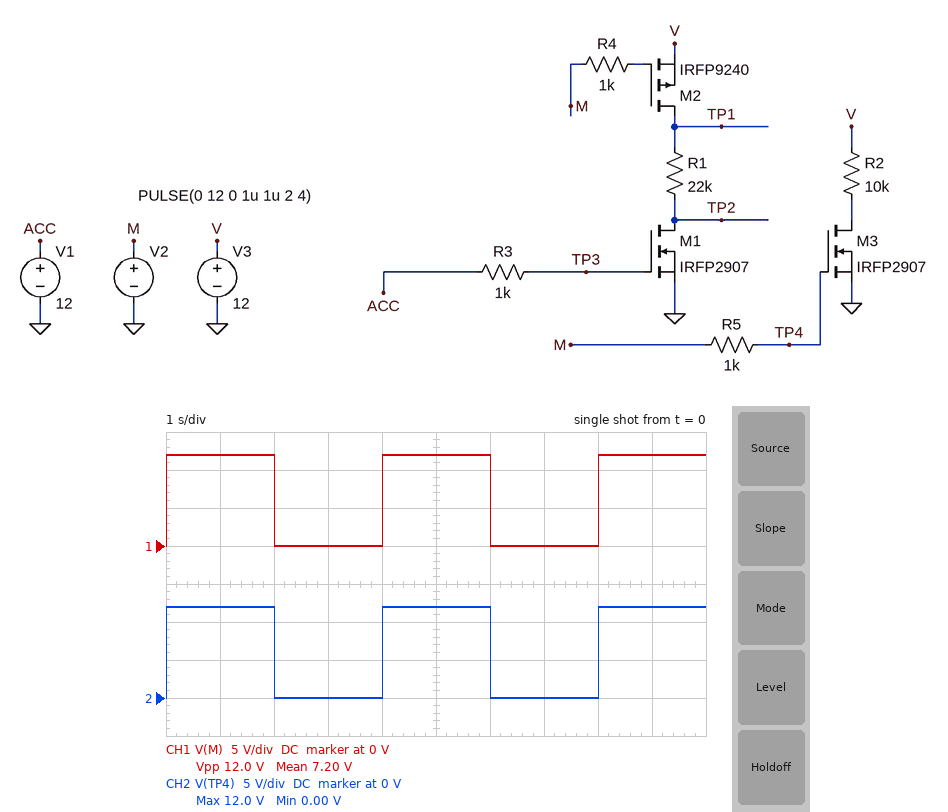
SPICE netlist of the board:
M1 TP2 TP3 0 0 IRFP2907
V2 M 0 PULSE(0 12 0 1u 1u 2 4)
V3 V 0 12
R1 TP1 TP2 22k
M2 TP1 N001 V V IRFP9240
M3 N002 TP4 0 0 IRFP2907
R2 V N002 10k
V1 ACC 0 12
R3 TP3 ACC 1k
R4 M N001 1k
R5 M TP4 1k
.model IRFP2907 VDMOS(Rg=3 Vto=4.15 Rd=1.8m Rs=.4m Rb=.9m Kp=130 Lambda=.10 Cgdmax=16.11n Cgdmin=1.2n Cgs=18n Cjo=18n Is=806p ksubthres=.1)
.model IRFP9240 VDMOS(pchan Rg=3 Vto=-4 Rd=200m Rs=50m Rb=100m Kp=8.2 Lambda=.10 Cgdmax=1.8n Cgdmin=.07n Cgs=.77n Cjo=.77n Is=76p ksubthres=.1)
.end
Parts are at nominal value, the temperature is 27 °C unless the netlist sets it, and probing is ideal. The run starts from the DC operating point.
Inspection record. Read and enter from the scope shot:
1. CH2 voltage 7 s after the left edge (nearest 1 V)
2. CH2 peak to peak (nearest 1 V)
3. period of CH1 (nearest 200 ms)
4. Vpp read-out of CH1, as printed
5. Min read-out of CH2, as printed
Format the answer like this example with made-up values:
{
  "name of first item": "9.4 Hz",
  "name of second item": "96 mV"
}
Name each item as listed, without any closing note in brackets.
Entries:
{
  "CH2 voltage 7 s after the left edge": "0 V",
  "CH2 peak to peak": "12 V",
  "period of CH1": "4.0 s",
  "Vpp read-out of CH1, as printed": "12.0 V",
  "Min read-out of CH2, as printed": "0.00 V"
}
